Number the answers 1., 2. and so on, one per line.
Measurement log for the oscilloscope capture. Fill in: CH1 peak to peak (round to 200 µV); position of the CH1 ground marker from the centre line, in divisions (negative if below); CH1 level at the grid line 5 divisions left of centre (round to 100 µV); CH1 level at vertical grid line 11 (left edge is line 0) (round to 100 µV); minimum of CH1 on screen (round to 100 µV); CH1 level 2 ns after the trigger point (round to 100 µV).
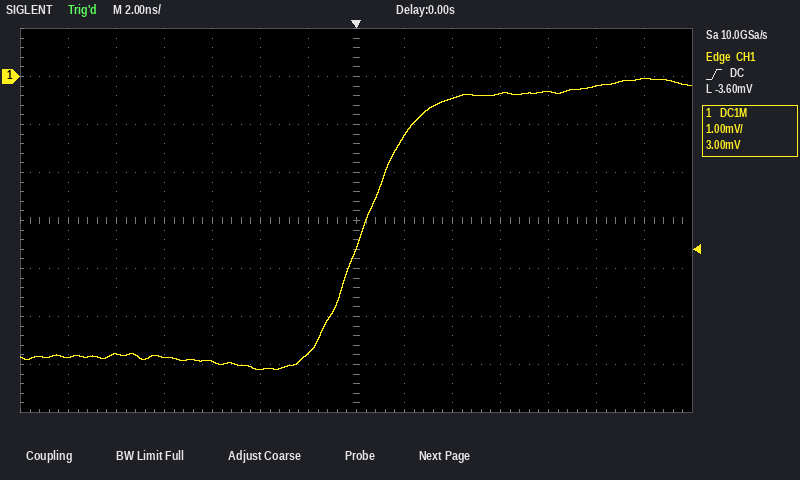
1. 6.0 mV
2. +3.0 div
3. -5.8 mV
4. -300 µV
5. -6.1 mV
6. -1.2 mV
